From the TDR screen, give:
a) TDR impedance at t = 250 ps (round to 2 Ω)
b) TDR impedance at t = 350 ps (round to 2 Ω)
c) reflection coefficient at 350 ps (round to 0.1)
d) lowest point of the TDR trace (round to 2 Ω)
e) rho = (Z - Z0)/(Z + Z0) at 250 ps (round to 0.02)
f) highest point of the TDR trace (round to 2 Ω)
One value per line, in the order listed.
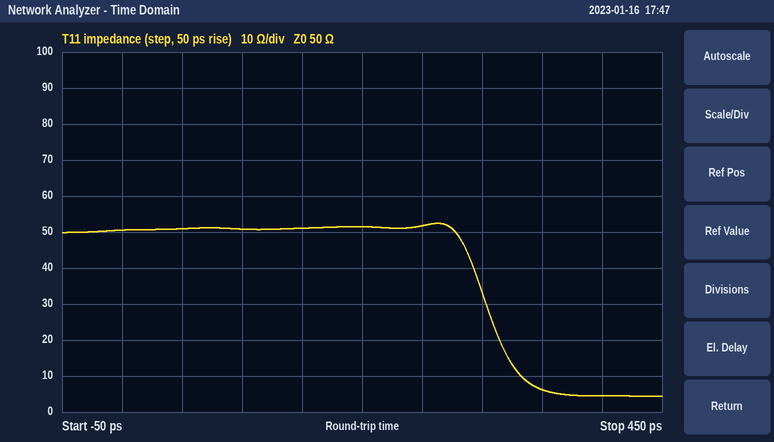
52 Ω
6 Ω
-0.8
4 Ω
+0.02
52 Ω
